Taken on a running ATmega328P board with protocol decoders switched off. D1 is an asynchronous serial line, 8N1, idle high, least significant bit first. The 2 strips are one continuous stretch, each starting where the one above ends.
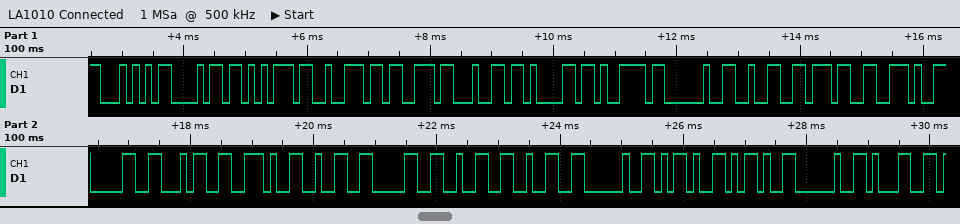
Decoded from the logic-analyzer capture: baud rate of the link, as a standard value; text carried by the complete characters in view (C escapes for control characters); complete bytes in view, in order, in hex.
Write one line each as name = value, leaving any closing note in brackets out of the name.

baud rate of the link, as a standard value = 9600 baud
text carried by the complete characters in view = "Thursday 27.04.2022 -- 1"
complete bytes in view, in order, in hex = 54 68 75 72 73 64 61 79 20 32 37 2E 30 34 2E 32 30 32 32 20 2D 2D 20 31
